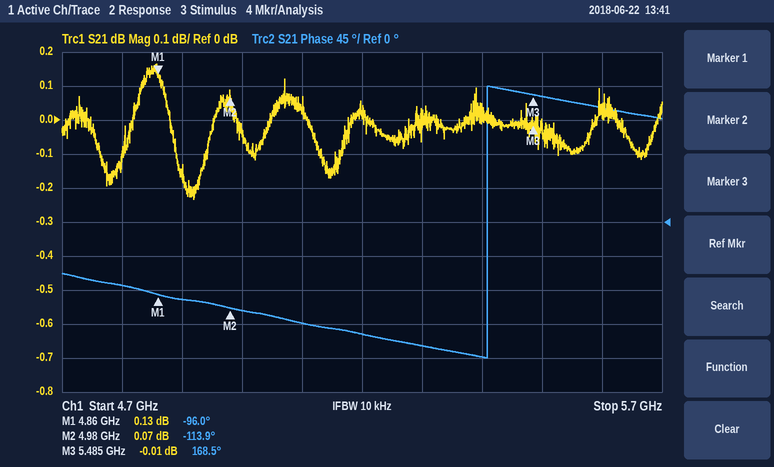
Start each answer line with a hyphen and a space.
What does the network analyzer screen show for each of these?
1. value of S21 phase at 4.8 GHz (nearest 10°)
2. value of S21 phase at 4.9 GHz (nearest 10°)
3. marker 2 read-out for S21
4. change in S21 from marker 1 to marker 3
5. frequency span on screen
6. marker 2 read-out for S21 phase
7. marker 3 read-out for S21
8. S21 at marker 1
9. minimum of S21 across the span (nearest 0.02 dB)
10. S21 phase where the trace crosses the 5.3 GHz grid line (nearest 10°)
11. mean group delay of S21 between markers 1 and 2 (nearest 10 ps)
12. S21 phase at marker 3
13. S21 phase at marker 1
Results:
- -80°
- -100°
- 0.07 dB
- -0.14 dB
- 1 GHz
- -113.9°
- -0.01 dB
- 0.13 dB
- -0.24 dB
- -160°
- 410 ps
- 168.5°
- -96.0°
